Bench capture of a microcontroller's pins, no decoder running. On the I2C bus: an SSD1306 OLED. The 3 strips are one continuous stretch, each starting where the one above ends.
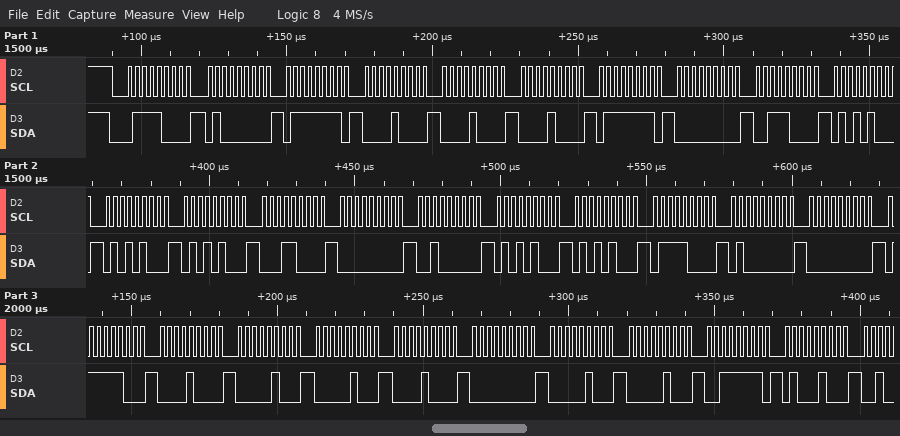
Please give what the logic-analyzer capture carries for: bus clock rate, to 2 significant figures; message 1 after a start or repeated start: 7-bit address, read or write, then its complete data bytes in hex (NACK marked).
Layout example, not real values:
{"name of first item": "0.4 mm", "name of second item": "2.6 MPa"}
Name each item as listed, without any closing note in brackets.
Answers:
{"bus clock rate, to 2 significant figures": "400 kHz", "message 1 after a start or repeated start: 7-bit address, read or write, then its complete data bytes in hex": "0x3C write: 40 7F 08 08 08 7F 00 38 54 54 54 18 00 20 54 54 78 40 00 7C 08 04 04 08 00 04 04 3F 44"}
